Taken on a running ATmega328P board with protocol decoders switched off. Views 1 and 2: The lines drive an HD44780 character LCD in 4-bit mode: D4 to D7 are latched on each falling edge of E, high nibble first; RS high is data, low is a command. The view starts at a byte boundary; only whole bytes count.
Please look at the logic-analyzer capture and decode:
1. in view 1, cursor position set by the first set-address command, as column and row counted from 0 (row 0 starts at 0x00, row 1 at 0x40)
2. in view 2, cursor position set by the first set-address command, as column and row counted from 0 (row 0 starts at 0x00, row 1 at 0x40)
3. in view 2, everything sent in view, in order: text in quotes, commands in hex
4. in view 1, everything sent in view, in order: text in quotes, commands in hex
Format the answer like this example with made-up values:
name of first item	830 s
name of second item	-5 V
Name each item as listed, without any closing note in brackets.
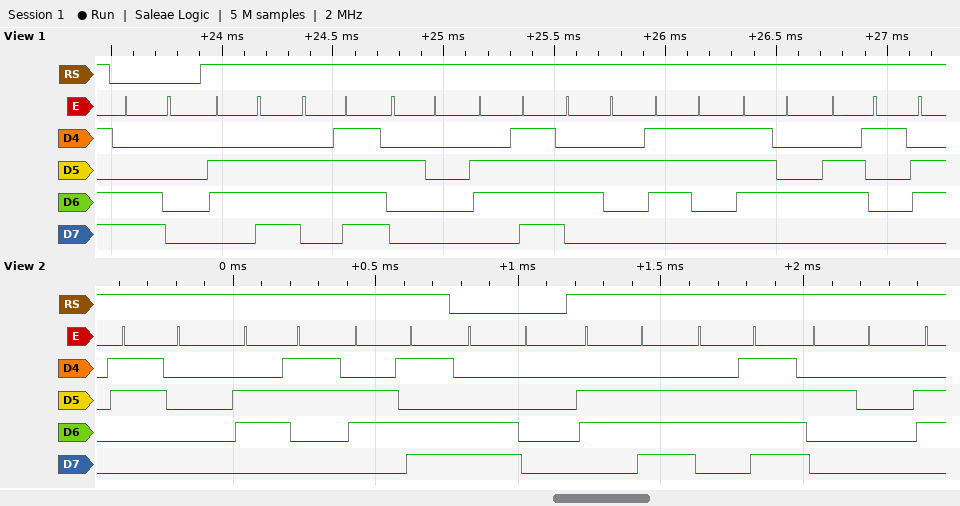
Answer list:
in view 1, cursor position set by the first set-address command, as column and row counted from 0	column 0, row 1
in view 2, cursor position set by the first set-address command, as column and row counted from 0	column 0, row 1
in view 2, everything sent in view, in order: text in quotes, commands in hex	"0cm" 0xC0 "no "
in view 1, everything sent in view, in order: text in quotes, commands in hex	0xC0 "no obsta"
